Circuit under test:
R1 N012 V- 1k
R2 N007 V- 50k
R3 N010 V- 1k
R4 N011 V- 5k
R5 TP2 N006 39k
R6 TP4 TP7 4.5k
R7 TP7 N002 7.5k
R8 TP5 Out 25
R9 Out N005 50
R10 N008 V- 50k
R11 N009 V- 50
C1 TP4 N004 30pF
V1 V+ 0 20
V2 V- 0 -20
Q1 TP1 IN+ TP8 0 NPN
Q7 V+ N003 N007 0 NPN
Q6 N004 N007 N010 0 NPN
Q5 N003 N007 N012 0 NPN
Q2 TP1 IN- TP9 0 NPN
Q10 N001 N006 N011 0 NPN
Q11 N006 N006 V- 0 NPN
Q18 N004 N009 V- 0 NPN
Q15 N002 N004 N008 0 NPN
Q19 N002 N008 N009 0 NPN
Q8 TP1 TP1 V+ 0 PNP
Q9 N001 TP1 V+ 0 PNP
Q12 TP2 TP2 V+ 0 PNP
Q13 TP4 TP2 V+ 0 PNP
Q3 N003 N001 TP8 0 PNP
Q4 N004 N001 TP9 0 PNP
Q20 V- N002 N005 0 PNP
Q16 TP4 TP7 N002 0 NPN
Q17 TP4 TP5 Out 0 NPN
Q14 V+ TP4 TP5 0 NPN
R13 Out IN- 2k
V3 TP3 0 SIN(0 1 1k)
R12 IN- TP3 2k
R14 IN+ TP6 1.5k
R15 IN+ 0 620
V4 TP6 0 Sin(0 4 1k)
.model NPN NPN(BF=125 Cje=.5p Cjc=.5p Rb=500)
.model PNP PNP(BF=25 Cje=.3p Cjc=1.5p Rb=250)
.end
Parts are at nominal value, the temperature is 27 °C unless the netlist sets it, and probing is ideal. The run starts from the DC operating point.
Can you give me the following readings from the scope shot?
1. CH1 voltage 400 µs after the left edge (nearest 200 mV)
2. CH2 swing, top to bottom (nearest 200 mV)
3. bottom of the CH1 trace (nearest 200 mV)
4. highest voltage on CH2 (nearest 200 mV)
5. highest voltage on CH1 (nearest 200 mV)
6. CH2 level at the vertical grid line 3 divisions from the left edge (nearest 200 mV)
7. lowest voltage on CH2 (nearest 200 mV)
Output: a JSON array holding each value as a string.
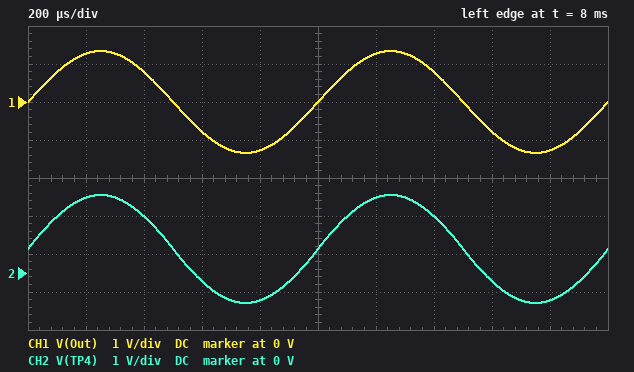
["800 mV", "2.8 V", "-1.4 V", "2.0 V", "1.4 V", "-200 mV", "-800 mV"]
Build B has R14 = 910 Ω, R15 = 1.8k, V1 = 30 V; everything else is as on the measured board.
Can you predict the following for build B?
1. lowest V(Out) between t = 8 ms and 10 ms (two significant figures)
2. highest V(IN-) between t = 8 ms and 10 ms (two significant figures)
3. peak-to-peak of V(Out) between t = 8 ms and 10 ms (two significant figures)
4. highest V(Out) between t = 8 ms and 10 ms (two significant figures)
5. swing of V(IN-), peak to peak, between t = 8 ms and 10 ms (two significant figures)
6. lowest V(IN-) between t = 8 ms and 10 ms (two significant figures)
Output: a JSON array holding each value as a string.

["-4.3 V", "2.7 V", "8.6 V", "4.3 V", "5.3 V", "-2.7 V"]
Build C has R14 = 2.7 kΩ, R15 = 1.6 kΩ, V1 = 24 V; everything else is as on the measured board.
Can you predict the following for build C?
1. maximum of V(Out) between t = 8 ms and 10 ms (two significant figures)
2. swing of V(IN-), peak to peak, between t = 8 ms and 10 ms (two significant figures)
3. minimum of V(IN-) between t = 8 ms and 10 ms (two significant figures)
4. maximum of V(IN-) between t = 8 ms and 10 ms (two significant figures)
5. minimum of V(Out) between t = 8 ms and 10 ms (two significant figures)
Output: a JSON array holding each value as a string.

["2.0 V", "3.0 V", "-1.5 V", "1.5 V", "-2.0 V"]
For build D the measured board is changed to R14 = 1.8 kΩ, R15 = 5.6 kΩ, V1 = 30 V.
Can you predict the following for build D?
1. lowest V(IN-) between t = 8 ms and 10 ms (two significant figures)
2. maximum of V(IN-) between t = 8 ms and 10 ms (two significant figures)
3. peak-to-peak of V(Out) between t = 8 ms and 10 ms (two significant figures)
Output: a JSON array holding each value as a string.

["-3.0 V", "3.0 V", "10 V"]
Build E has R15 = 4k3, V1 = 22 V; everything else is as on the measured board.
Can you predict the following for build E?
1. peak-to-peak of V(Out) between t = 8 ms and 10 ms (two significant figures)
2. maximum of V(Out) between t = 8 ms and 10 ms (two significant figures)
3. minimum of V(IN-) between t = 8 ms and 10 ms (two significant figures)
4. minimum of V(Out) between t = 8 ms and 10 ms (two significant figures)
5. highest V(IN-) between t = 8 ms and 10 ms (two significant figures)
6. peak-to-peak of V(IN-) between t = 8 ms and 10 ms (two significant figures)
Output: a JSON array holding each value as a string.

["9.9 V", "4.9 V", "-3.0 V", "-4.9 V", "3.0 V", "5.9 V"]
